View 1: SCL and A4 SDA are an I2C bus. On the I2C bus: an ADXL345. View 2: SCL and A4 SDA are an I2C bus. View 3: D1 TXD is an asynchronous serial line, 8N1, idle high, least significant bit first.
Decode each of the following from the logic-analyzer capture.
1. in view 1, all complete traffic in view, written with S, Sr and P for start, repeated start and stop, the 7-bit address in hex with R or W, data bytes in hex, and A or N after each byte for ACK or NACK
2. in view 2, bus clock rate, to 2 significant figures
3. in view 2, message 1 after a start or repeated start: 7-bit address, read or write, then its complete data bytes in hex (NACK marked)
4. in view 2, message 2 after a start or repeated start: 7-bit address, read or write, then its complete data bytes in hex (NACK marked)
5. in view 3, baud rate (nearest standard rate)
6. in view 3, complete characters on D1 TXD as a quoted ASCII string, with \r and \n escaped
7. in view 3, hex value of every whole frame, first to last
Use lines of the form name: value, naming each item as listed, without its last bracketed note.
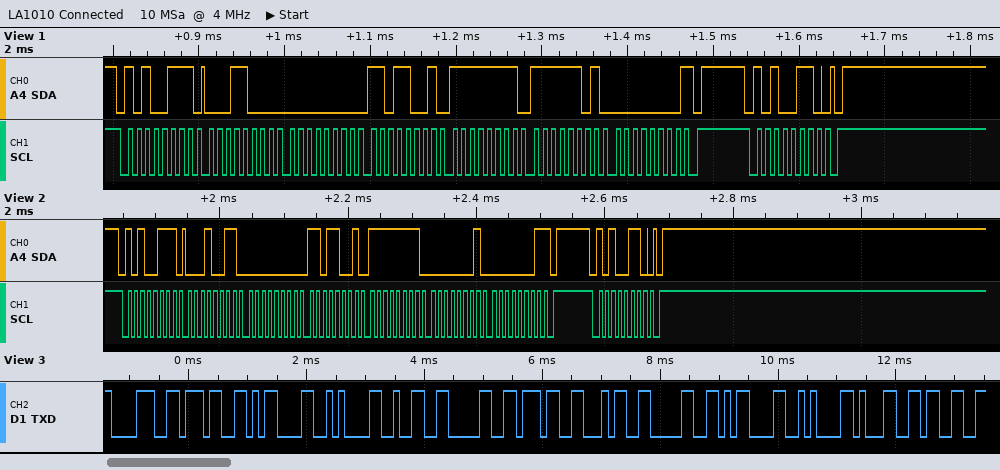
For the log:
in view 1, all complete traffic in view, written with S, Sr and P for start, repeated start and stop, the 7-bit address in hex with R or W, data bytes in hex, and A or N after each byte for ACK or NACK: S 53R A 18 A 00 A D9 A FF A FD A 00 N P S 53W A P
in view 2, bus clock rate, to 2 significant figures: 100 kHz
in view 2, message 1 after a start or repeated start: 7-bit address, read or write, then its complete data bytes in hex: 0x53 read: 13 00 D9 FF 01 01 NACK
in view 2, message 2 after a start or repeated start: 7-bit address, read or write, then its complete data bytes in hex: 0x53 write
in view 3, baud rate: 9600 baud
in view 3, complete characters on D1 TXD as a quoted ASCII string, with \r and \n escaped: "87\r\n20740\r\n13"
in view 3, hex value of every whole frame, first to last: 38 37 0D 0A 32 30 37 34 30 0D 0A 31 33
